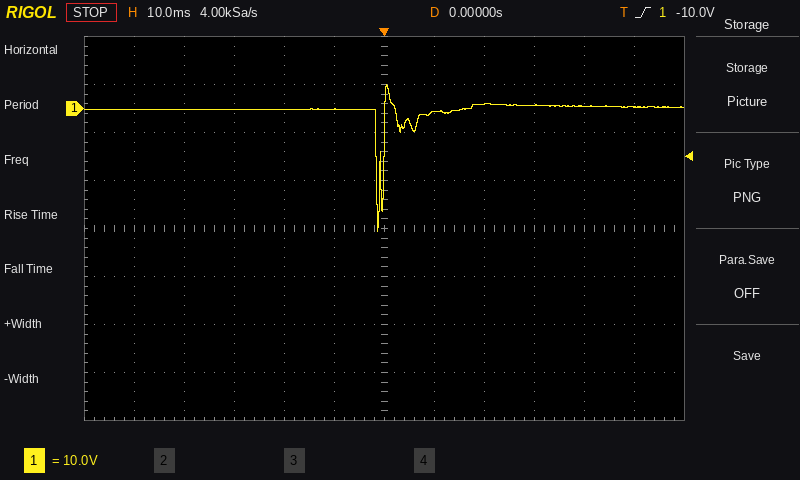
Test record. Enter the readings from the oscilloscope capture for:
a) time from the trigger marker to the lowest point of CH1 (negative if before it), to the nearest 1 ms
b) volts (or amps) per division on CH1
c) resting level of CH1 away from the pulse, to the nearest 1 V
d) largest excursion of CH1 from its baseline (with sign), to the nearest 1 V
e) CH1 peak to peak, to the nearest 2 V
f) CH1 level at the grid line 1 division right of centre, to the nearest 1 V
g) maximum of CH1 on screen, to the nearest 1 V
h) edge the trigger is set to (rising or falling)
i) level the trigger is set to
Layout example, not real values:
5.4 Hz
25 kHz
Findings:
-1 ms
10 V
0 V
-25 V
30 V
-1 V
5 V
rising
-10.0 V
